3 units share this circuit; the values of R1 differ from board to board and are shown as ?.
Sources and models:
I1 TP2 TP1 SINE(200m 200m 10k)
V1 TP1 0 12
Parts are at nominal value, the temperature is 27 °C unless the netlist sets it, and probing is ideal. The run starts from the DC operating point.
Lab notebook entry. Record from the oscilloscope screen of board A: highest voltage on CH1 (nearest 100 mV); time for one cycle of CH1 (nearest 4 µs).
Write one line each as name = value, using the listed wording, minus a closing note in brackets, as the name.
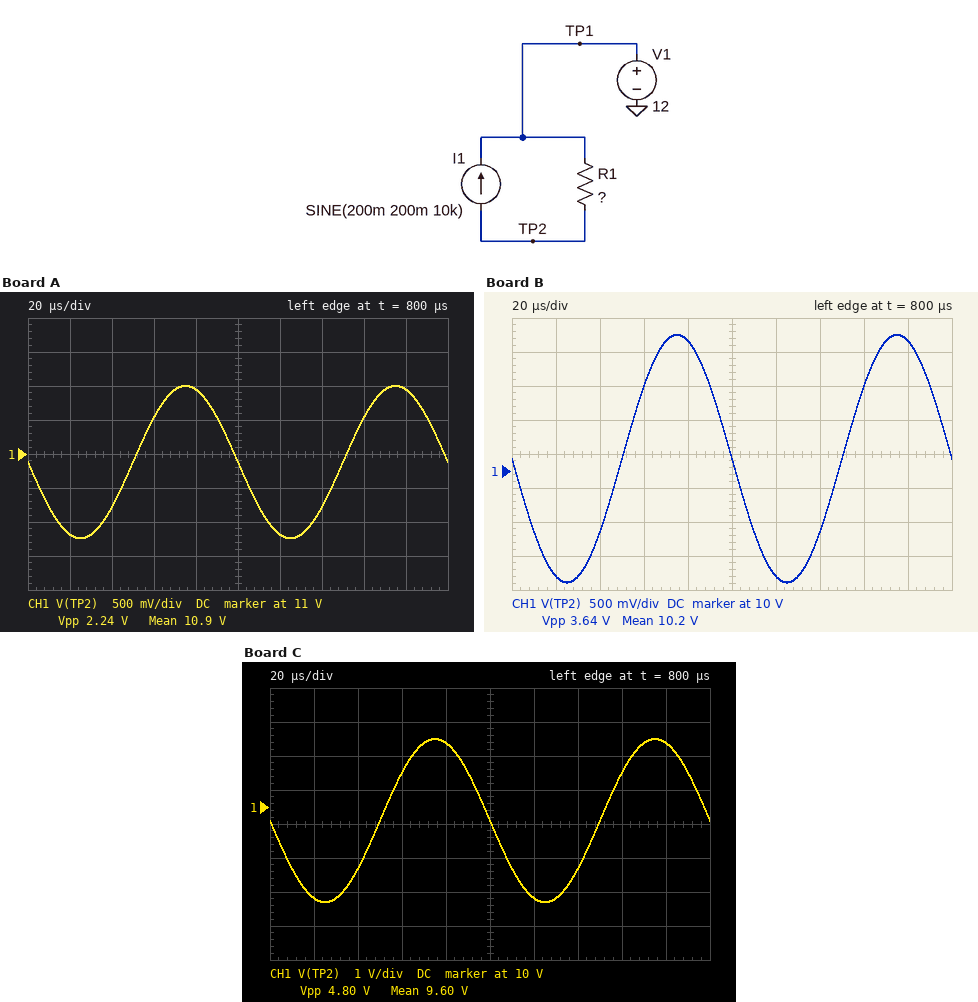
highest voltage on CH1 = 12.0 V
time for one cycle of CH1 = 100 µs
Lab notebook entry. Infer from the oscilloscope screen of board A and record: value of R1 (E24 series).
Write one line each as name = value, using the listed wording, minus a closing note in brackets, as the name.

value of R1 = 5.6 Ω
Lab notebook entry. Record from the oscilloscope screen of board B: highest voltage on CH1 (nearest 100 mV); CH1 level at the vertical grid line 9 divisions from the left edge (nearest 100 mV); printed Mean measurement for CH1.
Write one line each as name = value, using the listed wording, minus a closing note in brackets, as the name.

highest voltage on CH1 = 12.0 V
CH1 level at the vertical grid line 9 divisions from the left edge = 11.9 V
printed Mean measurement for CH1 = 10.2 V
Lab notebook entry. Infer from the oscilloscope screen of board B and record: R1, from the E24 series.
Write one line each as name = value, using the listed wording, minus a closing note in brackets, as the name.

R1, from the E24 series = 9.1 Ω
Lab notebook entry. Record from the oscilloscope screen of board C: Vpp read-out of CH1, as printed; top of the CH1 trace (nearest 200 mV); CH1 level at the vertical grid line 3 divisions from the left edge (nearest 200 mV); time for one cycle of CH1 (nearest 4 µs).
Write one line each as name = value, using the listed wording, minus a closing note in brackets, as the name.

Vpp read-out of CH1, as printed = 4.80 V
top of the CH1 trace = 12.0 V
CH1 level at the vertical grid line 3 divisions from the left edge = 11.0 V
time for one cycle of CH1 = 100 µs
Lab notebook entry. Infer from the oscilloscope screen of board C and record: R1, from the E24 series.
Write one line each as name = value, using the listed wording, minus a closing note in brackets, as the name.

R1, from the E24 series = 12 Ω
